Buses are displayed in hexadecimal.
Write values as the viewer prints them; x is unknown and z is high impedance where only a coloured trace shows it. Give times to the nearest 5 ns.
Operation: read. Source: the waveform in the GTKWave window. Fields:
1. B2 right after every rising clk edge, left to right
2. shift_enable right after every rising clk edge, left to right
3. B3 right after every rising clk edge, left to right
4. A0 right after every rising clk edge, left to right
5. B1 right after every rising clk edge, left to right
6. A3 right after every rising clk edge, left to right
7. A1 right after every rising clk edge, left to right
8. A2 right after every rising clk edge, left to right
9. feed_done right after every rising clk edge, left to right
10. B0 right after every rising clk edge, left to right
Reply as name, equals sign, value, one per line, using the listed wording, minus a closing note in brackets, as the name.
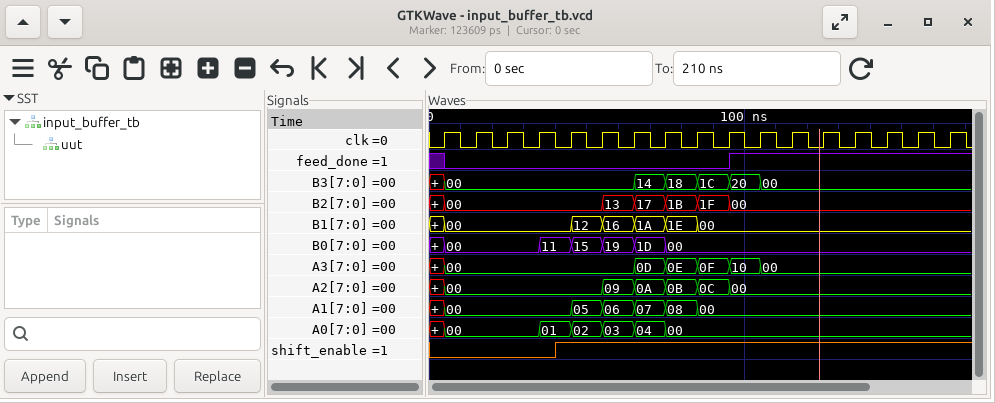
B2 right after every rising clk edge, left to right = 00, 00, 00, 00, 00, 13, 17, 1B, 1F, 00, 00, 00, 00, 00, 00, 00, 00
shift_enable right after every rising clk edge, left to right = 0 0 0 0 1 1 1 1 1 1 1 1 1 1 1 1 1
B3 right after every rising clk edge, left to right = 00, 00, 00, 00, 00, 00, 14, 18, 1C, 20, 00, 00, 00, 00, 00, 00, 00
A0 right after every rising clk edge, left to right = 00, 00, 00, 01, 02, 03, 04, 00, 00, 00, 00, 00, 00, 00, 00, 00, 00
B1 right after every rising clk edge, left to right = 00, 00, 00, 00, 12, 16, 1A, 1E, 00, 00, 00, 00, 00, 00, 00, 00, 00
A3 right after every rising clk edge, left to right = 00, 00, 00, 00, 00, 00, 0D, 0E, 0F, 10, 00, 00, 00, 00, 00, 00, 00
A1 right after every rising clk edge, left to right = 00, 00, 00, 00, 05, 06, 07, 08, 00, 00, 00, 00, 00, 00, 00, 00, 00
A2 right after every rising clk edge, left to right = 00, 00, 00, 00, 00, 09, 0A, 0B, 0C, 00, 00, 00, 00, 00, 00, 00, 00
feed_done right after every rising clk edge, left to right = 0 0 0 0 0 0 0 0 0 1 1 1 1 1 1 1 1
B0 right after every rising clk edge, left to right = 00, 00, 00, 11, 15, 19, 1D, 00, 00, 00, 00, 00, 00, 00, 00, 00, 00
